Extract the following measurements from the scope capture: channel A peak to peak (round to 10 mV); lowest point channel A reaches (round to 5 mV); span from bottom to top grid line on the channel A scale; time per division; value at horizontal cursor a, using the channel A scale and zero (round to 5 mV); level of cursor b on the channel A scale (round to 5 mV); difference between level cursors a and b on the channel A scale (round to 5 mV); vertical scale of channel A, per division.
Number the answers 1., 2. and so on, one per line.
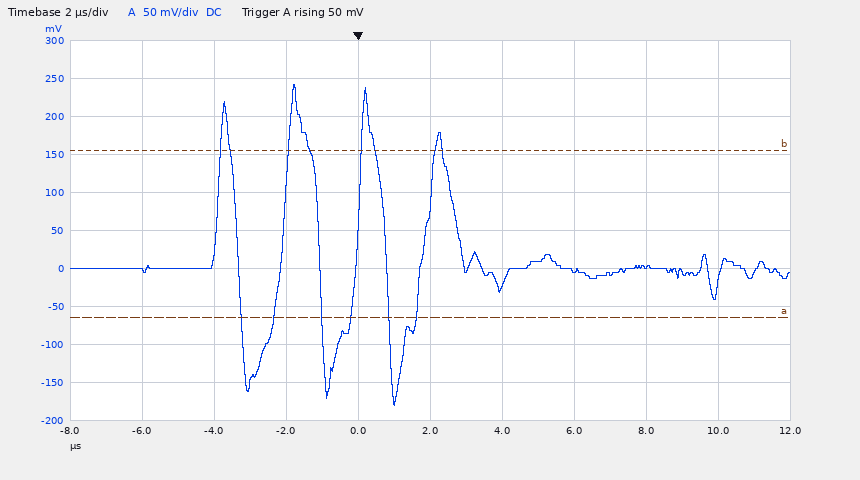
1. 420 mV
2. -180 mV
3. 500 mV
4. 2 µs
5. -65 mV
6. 155 mV
7. 220 mV
8. 50 mV
